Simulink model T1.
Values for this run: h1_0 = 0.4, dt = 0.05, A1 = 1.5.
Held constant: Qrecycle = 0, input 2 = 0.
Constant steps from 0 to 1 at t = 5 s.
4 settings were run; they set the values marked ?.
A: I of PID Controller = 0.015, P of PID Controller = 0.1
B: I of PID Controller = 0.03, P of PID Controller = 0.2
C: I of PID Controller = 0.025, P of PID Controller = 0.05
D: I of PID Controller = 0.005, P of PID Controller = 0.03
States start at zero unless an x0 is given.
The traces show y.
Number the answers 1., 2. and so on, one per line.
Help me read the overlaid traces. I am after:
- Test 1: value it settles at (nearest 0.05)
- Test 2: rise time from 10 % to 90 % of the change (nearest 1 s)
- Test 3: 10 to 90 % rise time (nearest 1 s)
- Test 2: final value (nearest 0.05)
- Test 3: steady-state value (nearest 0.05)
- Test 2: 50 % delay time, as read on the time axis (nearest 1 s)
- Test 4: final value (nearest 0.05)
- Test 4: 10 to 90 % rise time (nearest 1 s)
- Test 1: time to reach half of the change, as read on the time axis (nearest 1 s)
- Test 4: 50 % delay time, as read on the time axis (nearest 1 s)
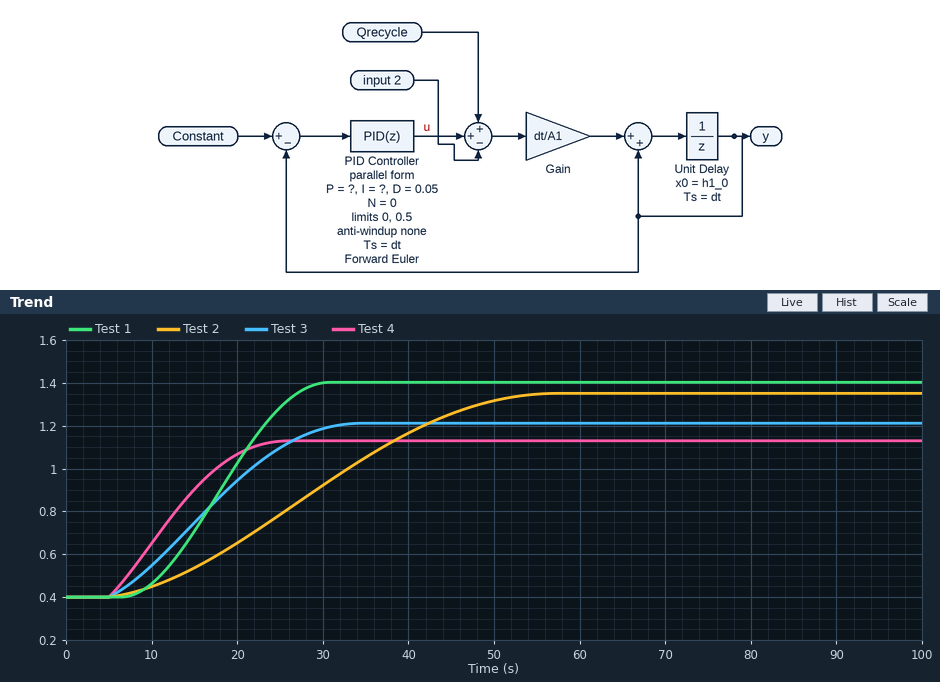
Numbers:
1. 1.40
2. 32 s
3. 18 s
4. 1.35
5. 1.20
6. 28 s
7. 1.15
8. 13 s
9. 18 s
10. 12 s
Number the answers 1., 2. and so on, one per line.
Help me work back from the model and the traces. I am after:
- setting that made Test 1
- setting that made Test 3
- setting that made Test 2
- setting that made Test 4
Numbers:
1. C
2. A
3. D
4. B
